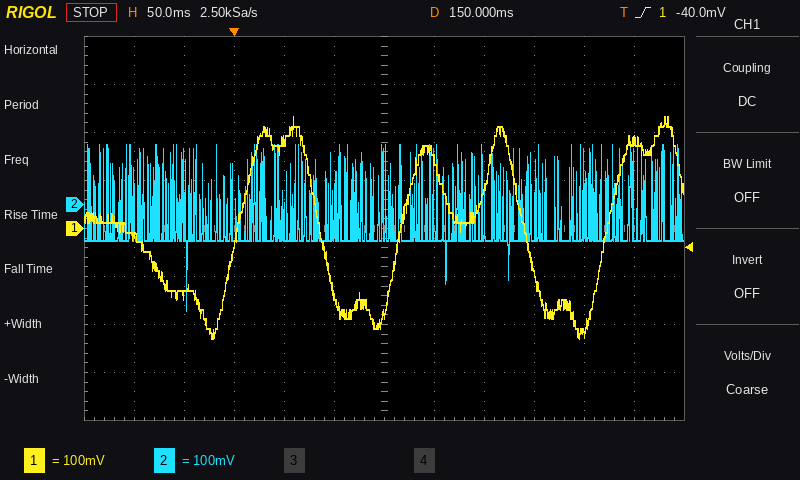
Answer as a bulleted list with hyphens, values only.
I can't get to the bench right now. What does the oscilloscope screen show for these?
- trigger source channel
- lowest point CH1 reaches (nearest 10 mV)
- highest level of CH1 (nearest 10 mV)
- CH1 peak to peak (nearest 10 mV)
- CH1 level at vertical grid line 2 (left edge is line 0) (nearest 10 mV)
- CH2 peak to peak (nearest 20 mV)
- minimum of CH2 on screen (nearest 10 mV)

- CH1
- -230 mV
- 230 mV
- 460 mV
- -140 mV
- 340 mV
- -220 mV
